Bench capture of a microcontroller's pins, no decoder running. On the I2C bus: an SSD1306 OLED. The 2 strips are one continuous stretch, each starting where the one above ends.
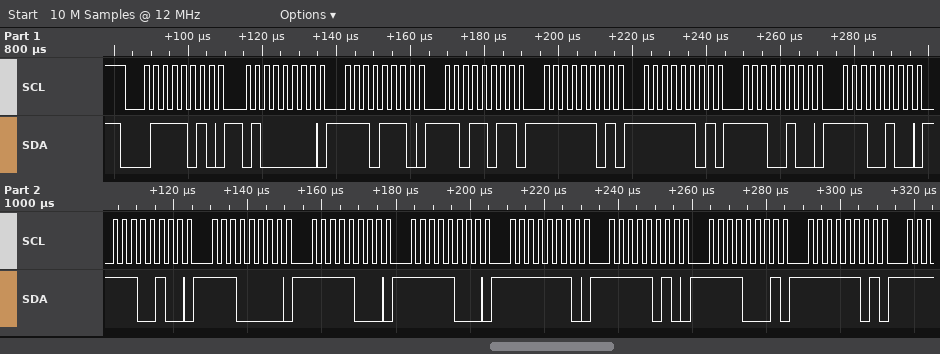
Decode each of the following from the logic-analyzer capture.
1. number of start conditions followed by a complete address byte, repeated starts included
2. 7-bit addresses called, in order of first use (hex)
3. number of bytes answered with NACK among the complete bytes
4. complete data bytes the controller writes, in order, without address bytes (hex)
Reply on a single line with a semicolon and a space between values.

1; 0x3D; 0; 40 EE DB FD FD E4 E4 E4 E0 F8 F8 FE FA F1 FD
